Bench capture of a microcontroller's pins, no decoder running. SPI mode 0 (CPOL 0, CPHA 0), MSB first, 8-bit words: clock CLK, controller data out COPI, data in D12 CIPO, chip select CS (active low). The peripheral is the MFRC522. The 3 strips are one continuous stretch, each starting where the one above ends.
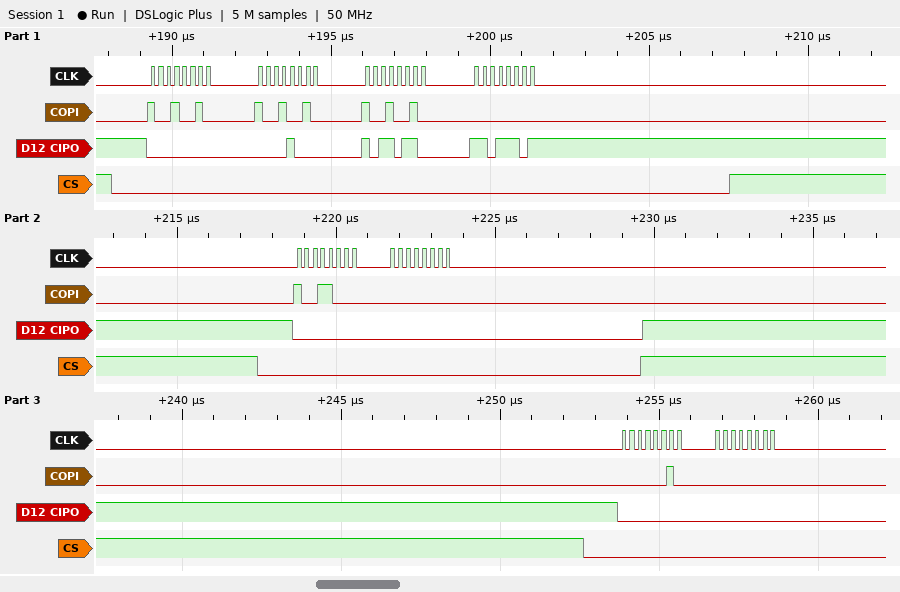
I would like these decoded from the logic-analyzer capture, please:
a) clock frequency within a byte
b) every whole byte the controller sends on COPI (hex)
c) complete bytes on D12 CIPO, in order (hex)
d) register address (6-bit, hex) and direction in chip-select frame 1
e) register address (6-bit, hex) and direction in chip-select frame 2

4 MHz
0x92 0x92 0x92 0x00 0x98 0x00 0x02 0x00
0x00 0x08 0xB6 0xDD 0x00 0x00 0x00 0x00
0x09 read
0x0C read
